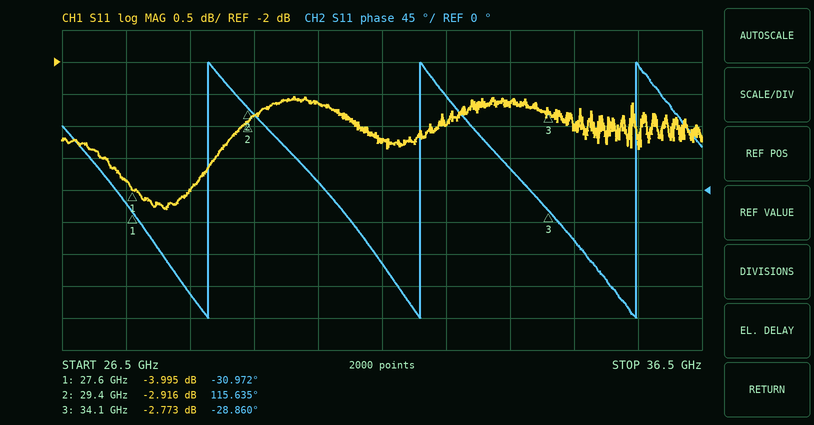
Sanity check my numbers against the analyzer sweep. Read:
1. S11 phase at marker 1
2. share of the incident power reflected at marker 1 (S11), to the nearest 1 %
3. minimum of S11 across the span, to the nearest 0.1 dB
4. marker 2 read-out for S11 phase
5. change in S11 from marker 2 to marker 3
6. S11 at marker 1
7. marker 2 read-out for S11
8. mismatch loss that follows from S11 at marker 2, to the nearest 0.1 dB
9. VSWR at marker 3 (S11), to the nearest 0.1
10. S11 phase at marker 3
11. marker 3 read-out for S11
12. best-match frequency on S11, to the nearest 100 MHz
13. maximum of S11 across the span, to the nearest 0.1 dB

-30.972°
40 %
-4.3 dB
115.635°
0.143 dB
-3.995 dB
-2.916 dB
3.1 dB
6.3
-28.860°
-2.773 dB
28.1 GHz
-2.5 dB
